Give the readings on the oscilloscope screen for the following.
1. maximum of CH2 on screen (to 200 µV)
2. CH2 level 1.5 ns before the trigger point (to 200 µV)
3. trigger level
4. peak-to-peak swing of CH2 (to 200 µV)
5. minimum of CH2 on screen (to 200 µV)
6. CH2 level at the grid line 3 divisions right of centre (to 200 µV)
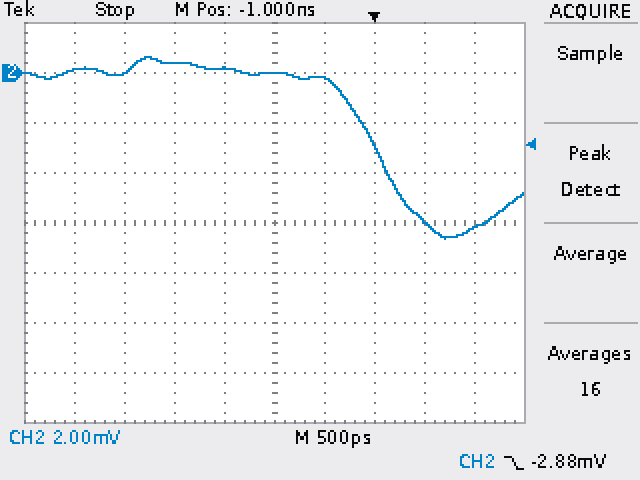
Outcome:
600 µV
200 µV
-2.88 mV
7.2 mV
-6.6 mV
-6.0 mV
